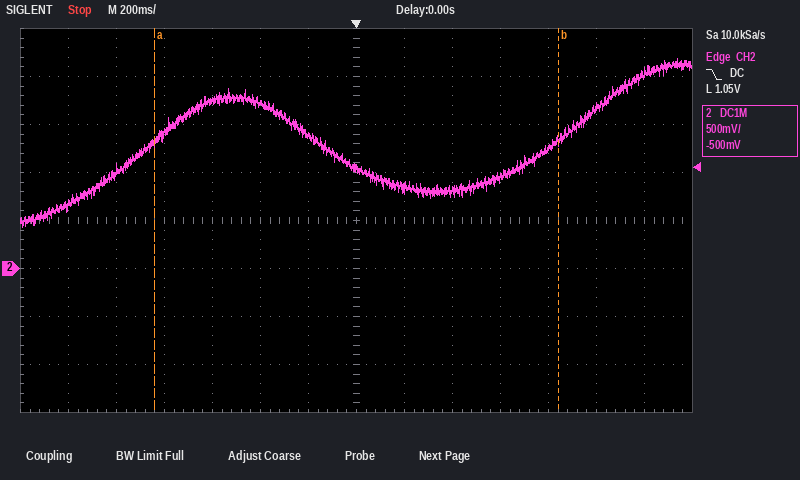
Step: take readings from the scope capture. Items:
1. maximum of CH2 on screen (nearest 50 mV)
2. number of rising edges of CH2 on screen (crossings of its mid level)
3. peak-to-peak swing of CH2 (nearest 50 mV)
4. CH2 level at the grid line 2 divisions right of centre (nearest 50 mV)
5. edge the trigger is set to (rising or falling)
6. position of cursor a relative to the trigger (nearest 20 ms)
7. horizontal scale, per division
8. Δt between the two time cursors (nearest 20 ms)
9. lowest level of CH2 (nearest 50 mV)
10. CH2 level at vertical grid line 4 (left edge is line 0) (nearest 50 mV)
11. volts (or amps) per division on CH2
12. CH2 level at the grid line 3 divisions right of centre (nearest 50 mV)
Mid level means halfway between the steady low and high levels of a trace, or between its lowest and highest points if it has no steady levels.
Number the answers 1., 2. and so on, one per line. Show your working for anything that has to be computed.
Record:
1. 2.20 V
2. 2
3. 2.20 V − (450 mV) = 1.75 V
4. 800 mV
5. falling
6. -840 ms
7. 200 ms
8. 1.68 s
9. 450 mV
10. 1.75 V
11. 500 mV
12. 950 mV
